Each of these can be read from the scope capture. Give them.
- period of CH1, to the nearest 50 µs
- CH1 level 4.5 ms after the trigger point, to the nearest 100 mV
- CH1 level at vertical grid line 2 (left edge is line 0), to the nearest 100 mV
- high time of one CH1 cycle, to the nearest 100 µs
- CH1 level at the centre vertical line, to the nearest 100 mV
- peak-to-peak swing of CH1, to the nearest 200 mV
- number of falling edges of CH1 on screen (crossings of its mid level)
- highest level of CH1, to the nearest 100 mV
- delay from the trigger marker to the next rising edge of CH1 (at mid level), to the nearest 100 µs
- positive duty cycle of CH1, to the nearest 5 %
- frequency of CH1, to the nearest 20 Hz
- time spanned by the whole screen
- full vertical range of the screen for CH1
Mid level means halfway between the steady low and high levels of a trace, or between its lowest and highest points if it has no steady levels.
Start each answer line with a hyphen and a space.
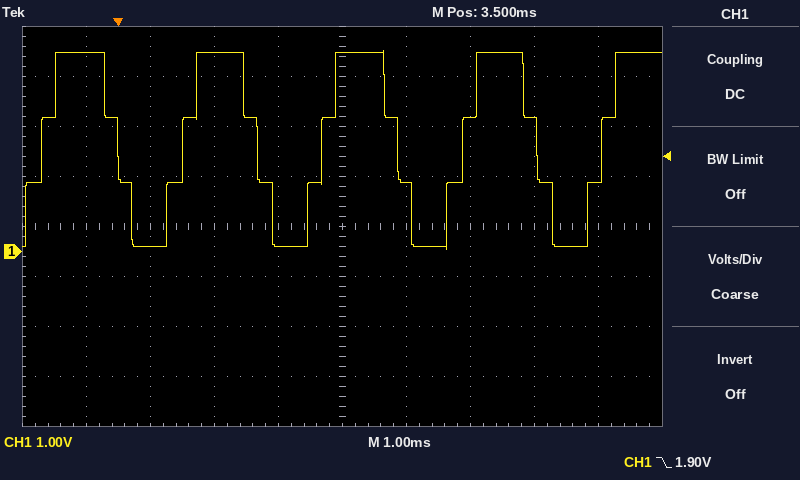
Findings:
- 2.20 ms
- 1.4 V
- 100 mV
- 1.2 ms
- 4.0 V
- 4.0 V
- 4
- 4.0 V
- 1.0 ms
- 55 %
- 460 Hz
- 10 ms
- 8 V
